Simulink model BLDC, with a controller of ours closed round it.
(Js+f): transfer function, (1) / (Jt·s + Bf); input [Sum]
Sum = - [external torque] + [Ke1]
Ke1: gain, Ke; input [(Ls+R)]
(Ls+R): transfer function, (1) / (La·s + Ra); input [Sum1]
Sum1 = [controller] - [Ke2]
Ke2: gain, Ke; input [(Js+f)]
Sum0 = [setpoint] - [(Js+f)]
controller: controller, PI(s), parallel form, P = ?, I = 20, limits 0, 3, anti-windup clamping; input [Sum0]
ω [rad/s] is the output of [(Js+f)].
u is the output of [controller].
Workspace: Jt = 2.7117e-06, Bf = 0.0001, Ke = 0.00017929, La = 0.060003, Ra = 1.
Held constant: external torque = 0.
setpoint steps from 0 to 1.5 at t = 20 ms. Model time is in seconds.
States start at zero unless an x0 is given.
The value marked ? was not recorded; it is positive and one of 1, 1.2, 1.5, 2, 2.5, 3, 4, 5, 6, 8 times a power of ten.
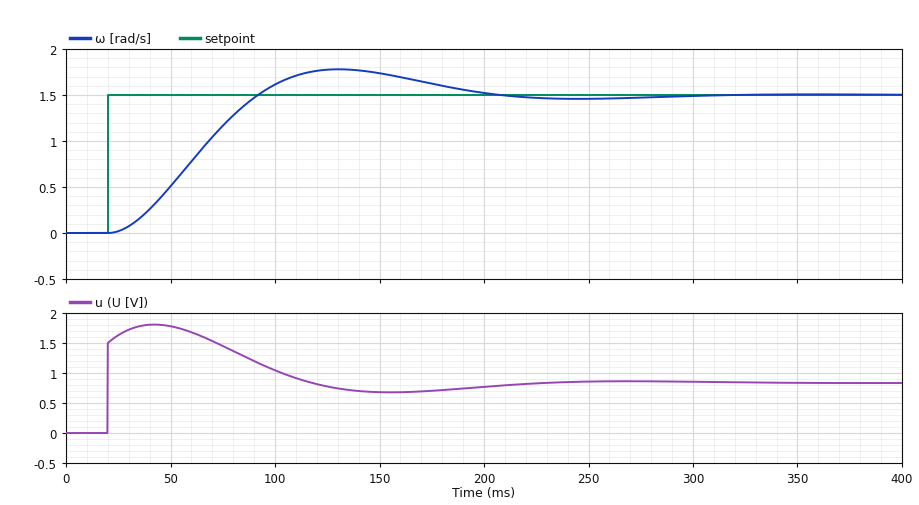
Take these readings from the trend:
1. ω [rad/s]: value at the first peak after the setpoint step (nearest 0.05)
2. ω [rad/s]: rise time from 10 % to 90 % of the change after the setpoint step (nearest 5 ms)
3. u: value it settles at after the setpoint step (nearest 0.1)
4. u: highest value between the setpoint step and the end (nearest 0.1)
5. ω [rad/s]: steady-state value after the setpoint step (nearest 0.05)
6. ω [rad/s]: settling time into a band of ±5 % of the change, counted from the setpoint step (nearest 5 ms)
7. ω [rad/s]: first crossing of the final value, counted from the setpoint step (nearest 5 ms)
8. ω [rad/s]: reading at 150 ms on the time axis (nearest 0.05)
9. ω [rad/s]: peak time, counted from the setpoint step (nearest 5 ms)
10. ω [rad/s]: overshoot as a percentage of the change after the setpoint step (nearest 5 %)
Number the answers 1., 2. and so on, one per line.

1. 1.80
2. 50 ms
3. 0.8
4. 1.8
5. 1.50
6. 165 ms
7. 70 ms
8. 1.75
9. 110 ms
10. 20 %
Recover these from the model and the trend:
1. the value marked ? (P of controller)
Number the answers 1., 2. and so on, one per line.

1. 1
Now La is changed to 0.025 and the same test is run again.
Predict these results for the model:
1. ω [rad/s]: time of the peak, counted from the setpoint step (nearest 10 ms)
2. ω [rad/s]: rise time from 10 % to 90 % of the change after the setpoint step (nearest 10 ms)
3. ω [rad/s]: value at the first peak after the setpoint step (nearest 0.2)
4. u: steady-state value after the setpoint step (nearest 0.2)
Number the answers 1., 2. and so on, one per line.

1. 70 ms
2. 40 ms
3. 1.6
4. 0.8
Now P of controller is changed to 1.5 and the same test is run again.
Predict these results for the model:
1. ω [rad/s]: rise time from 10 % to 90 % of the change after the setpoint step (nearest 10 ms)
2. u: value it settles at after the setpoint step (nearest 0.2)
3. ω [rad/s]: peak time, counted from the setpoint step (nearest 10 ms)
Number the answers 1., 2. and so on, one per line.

1. 40 ms
2. 0.8
3. 90 ms
